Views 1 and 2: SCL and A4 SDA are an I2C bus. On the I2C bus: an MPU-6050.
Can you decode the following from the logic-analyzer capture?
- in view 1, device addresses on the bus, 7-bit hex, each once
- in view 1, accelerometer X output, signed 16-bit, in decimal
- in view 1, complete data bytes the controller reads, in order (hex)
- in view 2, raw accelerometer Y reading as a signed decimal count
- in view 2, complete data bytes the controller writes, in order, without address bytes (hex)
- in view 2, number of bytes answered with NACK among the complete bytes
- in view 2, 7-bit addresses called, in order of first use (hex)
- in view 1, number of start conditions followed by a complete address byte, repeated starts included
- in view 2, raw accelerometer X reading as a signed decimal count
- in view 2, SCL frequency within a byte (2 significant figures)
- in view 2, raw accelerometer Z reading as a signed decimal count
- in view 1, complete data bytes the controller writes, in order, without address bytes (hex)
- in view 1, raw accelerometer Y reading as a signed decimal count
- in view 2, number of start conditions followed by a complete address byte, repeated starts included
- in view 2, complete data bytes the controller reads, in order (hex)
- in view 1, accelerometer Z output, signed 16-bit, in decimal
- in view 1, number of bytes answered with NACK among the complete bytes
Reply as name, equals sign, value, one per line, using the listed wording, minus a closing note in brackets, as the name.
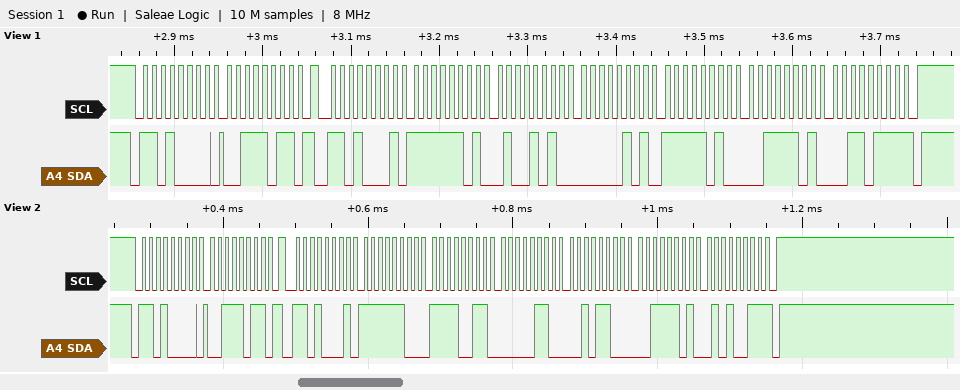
in view 1, device addresses on the bus, 7-bit hex, each once = 0x68
in view 1, accelerometer X output, signed 16-bit, in decimal = -694
in view 1, complete data bytes the controller reads, in order = FD 4A 05 FA 3D 37
in view 2, raw accelerometer Y reading as a signed decimal count = 1580
in view 2, complete data bytes the controller writes, in order, without address bytes = 3B
in view 2, number of bytes answered with NACK among the complete bytes = 1
in view 2, 7-bit addresses called, in order of first use = 0x68
in view 1, number of start conditions followed by a complete address byte, repeated starts included = 2
in view 2, raw accelerometer X reading as a signed decimal count = -781
in view 2, SCL frequency within a byte = 100 kHz
in view 2, raw accelerometer Z reading as a signed decimal count = 15699
in view 1, complete data bytes the controller writes, in order, without address bytes = 3B
in view 1, raw accelerometer Y reading as a signed decimal count = 1530
in view 2, number of start conditions followed by a complete address byte, repeated starts included = 2
in view 2, complete data bytes the controller reads, in order = FC F3 06 2C 3D 53
in view 1, accelerometer Z output, signed 16-bit, in decimal = 15671
in view 1, number of bytes answered with NACK among the complete bytes = 1
